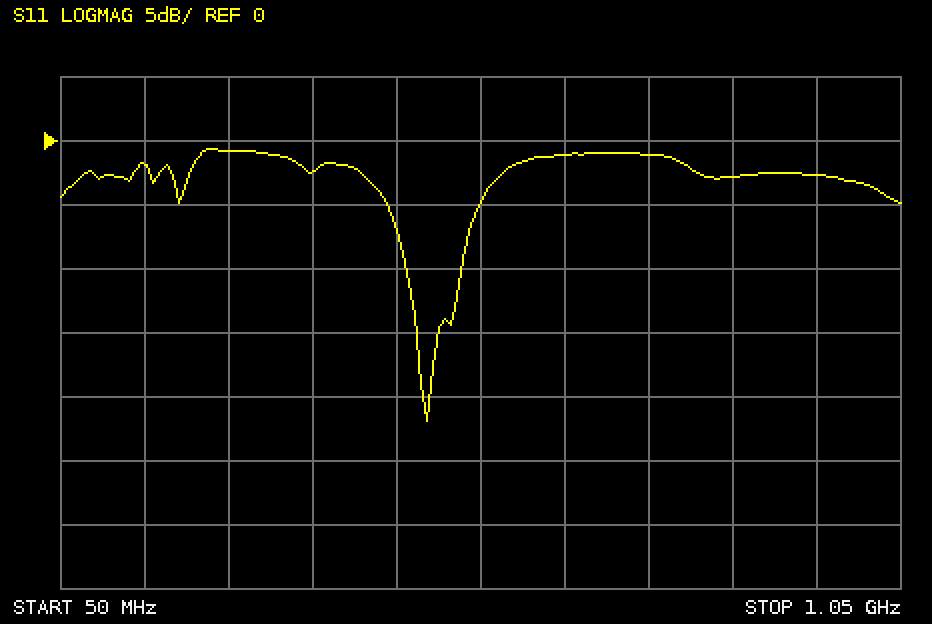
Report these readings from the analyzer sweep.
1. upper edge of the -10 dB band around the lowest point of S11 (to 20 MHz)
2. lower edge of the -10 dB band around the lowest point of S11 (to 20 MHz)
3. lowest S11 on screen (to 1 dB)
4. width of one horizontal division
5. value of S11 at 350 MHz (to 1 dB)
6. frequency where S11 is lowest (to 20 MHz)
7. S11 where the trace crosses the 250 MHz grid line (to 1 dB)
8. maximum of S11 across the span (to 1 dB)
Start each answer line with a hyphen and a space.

- 520 MHz
- 460 MHz
- -22 dB
- 100 MHz
- -2 dB
- 480 MHz
- -1 dB
- -1 dB
